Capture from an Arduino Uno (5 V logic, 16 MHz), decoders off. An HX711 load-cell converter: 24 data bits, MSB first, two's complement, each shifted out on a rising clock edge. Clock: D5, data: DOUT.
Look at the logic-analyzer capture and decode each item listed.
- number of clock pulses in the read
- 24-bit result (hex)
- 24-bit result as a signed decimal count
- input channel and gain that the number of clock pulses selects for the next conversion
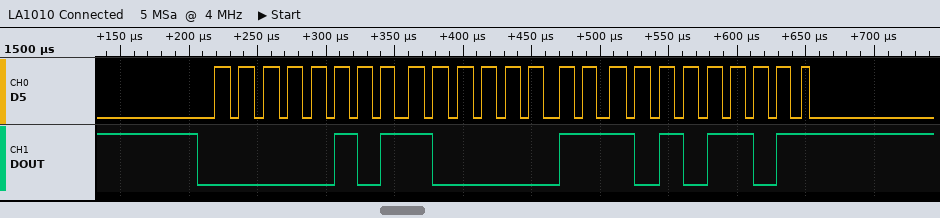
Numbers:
25
0x0583AD
361389
channel A, gain 128
